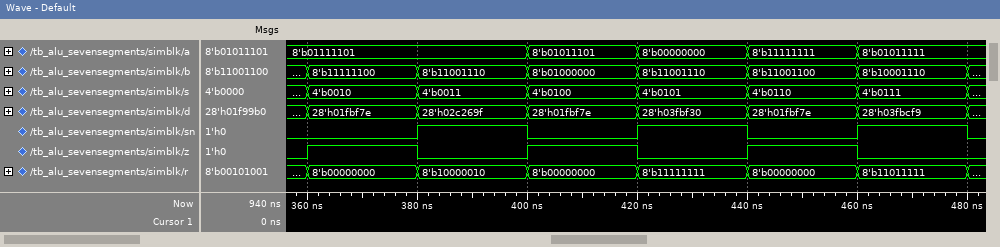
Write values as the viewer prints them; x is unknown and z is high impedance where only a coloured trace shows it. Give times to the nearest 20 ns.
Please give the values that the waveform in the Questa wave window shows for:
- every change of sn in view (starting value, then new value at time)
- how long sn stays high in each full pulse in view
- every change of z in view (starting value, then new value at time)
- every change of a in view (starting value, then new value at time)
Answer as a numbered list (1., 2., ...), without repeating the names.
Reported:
1. 0, 1 at 380 ns, 0 at 400 ns, 1 at 420 ns, 0 at 440 ns, 1 at 460 ns, 0 at 480 ns
2. 20 ns, 20 ns, 20 ns
3. 0, 1 at 360 ns, 0 at 380 ns, 1 at 400 ns, 0 at 420 ns, 1 at 440 ns, 0 at 460 ns
4. 8'b01111101, 8'b01011101 at 400 ns, 8'b00000000 at 420 ns, 8'b11111111 at 440 ns, 8'b01011111 at 460 ns
